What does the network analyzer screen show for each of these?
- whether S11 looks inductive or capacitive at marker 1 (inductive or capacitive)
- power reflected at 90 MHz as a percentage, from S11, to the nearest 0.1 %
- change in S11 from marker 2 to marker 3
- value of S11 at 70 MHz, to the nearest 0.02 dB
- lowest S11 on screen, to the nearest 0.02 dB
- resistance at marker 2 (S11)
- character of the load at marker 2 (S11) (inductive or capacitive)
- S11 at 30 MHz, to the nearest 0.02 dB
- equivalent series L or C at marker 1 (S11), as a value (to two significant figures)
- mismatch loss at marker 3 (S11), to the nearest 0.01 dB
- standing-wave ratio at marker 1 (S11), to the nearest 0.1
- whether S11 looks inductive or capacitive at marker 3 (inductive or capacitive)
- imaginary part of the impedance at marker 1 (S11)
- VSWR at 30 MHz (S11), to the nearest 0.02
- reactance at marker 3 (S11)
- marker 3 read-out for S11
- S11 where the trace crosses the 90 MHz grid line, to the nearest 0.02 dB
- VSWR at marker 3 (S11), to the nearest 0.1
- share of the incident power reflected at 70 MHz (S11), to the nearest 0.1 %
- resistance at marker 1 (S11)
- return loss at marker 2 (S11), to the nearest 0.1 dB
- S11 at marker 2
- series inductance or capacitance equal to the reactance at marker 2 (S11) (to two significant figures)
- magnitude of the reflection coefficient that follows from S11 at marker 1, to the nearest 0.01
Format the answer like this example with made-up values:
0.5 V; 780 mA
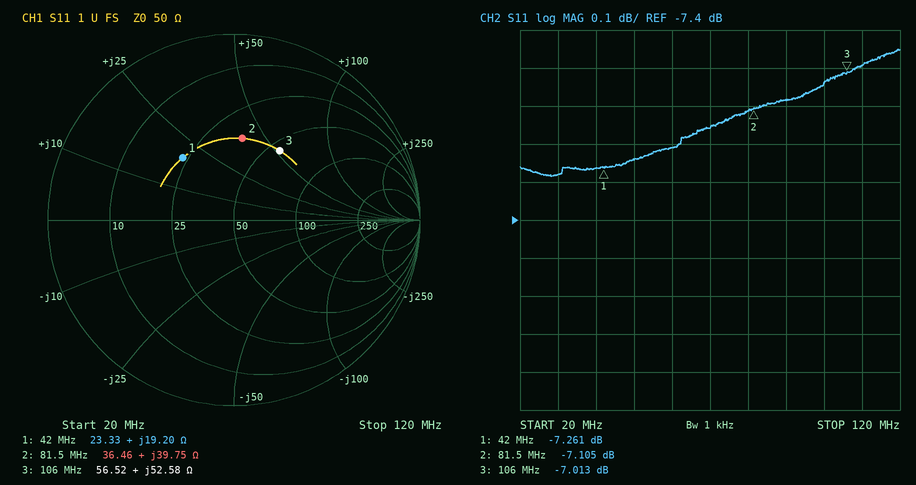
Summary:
inductive; 19.6 %; 0.092 dB; -7.16 dB; -7.28 dB; 36.46 Ω; inductive; -7.28 dB; 73 nH; 0.96 dB; 2.5; inductive; +19.20 Ω; 2.52; +52.58 Ω; -7.013 dB; -7.08 dB; 2.6; 19.2 %; 23.33 Ω; 7.1 dB; -7.105 dB; 78 nH; 0.43
